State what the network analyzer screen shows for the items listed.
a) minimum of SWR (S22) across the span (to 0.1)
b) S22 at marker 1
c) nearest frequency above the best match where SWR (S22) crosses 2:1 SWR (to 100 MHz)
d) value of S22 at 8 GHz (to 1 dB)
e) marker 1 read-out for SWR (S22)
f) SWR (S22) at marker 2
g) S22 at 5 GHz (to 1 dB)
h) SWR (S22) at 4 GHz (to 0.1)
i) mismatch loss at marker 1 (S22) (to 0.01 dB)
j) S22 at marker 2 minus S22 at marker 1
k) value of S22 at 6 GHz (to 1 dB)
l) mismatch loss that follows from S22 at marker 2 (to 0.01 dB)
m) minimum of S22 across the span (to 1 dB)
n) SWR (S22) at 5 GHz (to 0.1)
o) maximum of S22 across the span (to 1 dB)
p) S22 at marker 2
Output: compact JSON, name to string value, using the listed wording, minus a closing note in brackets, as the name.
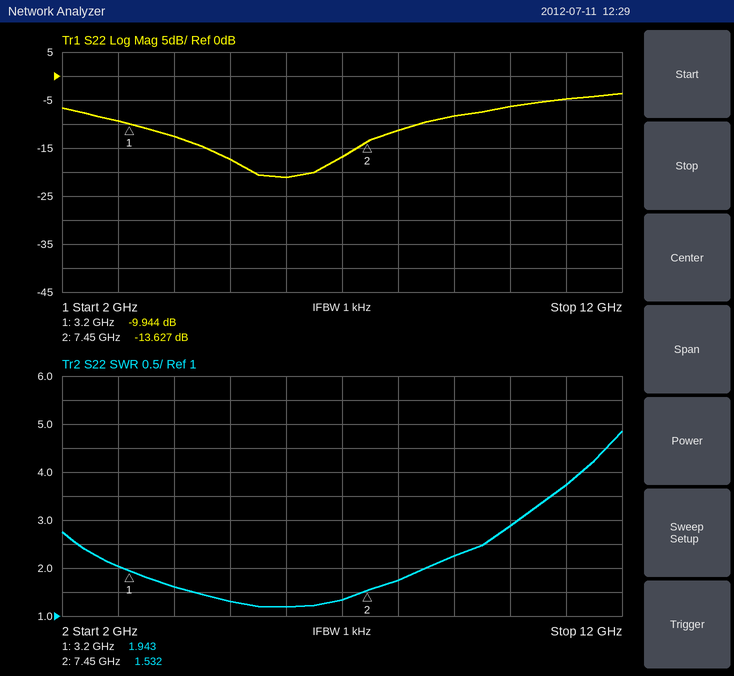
{"minimum of SWR (S22) across the span": "1.2", "S22 at marker 1": "-9.944 dB", "nearest frequency above the best match where SWR (S22) crosses 2:1 SWR": "8.5 GHz", "value of S22 at 8 GHz": "-11 dB", "marker 1 read-out for SWR": "1.943", "SWR (S22) at marker 2": "1.532", "S22 at 5 GHz": "-17 dB", "SWR (S22) at 4 GHz": "1.6", "mismatch loss at marker 1 (S22)": "0.46 dB", "S22 at marker 2 minus S22 at marker 1": "-3.683 dB", "value of S22 at 6 GHz": "-21 dB", "mismatch loss that follows from S22 at marker 2": "0.19 dB", "minimum of S22 across the span": "-21 dB", "SWR (S22) at 5 GHz": "1.3", "maximum of S22 across the span": "-4 dB", "S22 at marker 2": "-13.627 dB"}
